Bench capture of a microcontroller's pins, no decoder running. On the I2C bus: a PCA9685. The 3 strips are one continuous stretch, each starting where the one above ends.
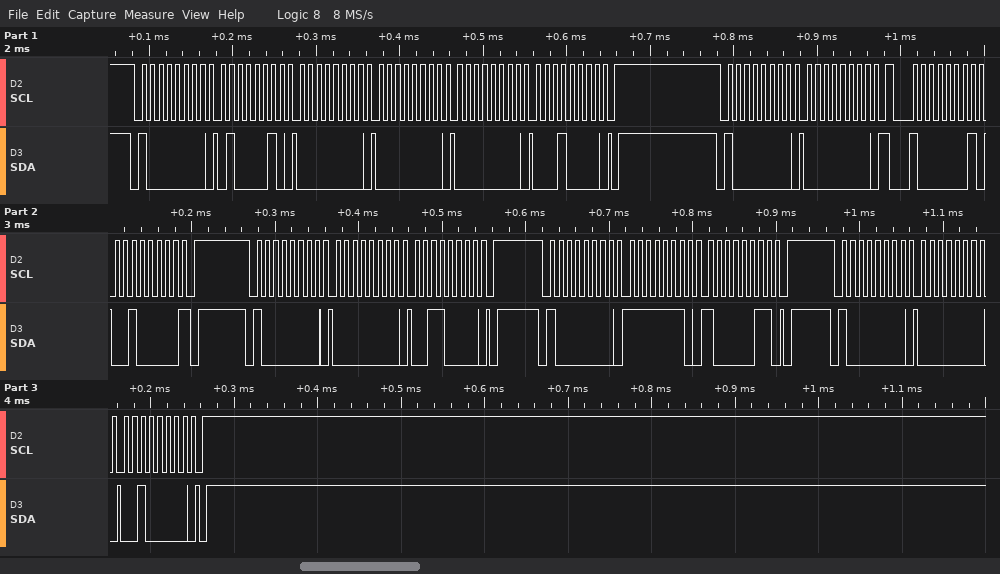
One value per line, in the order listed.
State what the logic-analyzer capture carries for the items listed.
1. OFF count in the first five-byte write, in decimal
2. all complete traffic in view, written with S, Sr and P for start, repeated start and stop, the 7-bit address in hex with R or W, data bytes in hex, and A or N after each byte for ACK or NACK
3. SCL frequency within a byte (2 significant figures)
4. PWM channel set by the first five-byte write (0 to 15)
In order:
4096
S 40W A 42 A 00 A 00 A 00 A 10 A P S 40W A 00 A Sr 40R A 20 N P S 40W A 00 A 30 A P S 40W A FE A 83 A P S 40W A 00 A 20 A P
100 kHz
15
